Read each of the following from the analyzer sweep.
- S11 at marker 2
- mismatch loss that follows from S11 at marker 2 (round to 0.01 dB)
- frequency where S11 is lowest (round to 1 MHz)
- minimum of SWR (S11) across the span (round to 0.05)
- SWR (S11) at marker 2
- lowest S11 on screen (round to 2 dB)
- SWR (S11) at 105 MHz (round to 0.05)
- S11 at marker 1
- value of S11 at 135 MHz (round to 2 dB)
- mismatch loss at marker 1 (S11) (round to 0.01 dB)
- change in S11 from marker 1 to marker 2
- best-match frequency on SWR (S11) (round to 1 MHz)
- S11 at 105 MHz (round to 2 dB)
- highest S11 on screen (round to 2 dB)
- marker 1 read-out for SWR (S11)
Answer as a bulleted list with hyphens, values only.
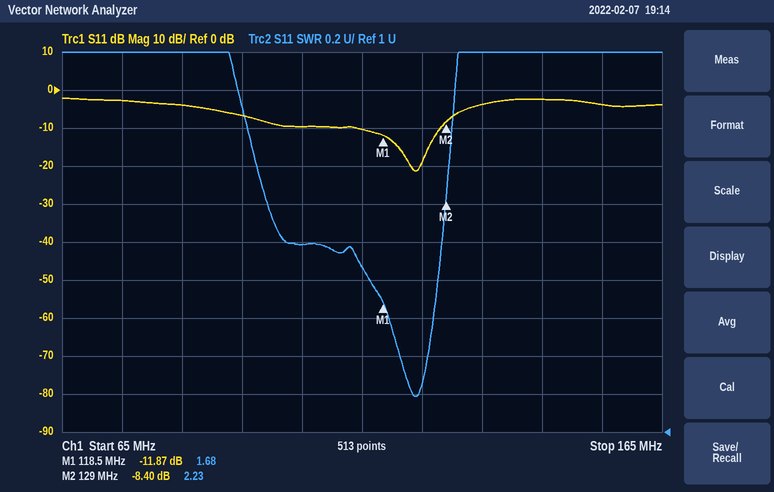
- -8.40 dB
- 0.68 dB
- 124 MHz
- 1.20
- 2.23
- -22 dB
- 2.00
- -11.87 dB
- -4 dB
- 0.29 dB
- 3.47 dB
- 124 MHz
- -10 dB
- -2 dB
- 1.68
